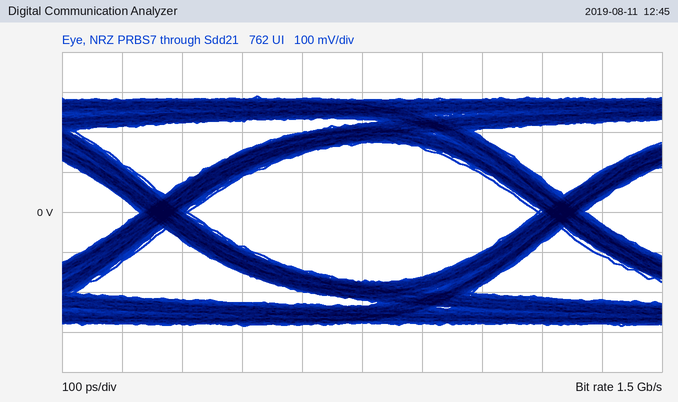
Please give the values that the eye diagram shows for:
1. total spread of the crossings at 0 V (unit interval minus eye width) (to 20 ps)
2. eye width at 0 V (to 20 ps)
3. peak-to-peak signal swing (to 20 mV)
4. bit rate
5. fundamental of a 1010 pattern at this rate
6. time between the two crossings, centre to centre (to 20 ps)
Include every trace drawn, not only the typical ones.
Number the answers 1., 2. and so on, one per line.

1. 80 ps
2. 580 ps
3. 580 mV
4. 1.5 Gb/s
5. 750 MHz
6. 660 ps
